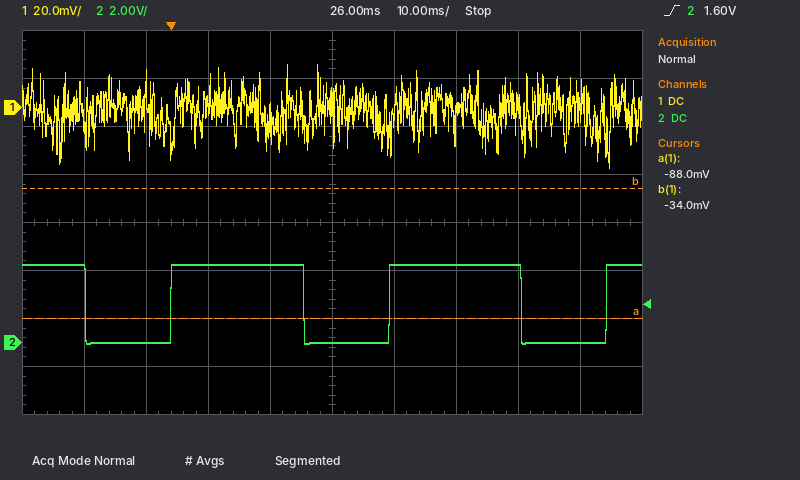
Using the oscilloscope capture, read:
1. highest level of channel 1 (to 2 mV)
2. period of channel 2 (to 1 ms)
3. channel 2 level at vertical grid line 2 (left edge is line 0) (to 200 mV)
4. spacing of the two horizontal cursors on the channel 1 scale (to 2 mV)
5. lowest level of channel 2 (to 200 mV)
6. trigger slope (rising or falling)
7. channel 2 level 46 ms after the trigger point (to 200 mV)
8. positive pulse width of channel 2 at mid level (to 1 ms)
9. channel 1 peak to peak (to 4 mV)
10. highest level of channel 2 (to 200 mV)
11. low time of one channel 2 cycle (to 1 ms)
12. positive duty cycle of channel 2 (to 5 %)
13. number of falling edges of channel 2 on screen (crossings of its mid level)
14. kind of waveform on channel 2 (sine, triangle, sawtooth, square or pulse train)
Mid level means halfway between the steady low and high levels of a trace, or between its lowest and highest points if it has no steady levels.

18 mV
35 ms
0.0 V
54 mV
0.0 V
rising
3.2 V
21 ms
44 mV
3.2 V
14 ms
60 %
3
pulse train
